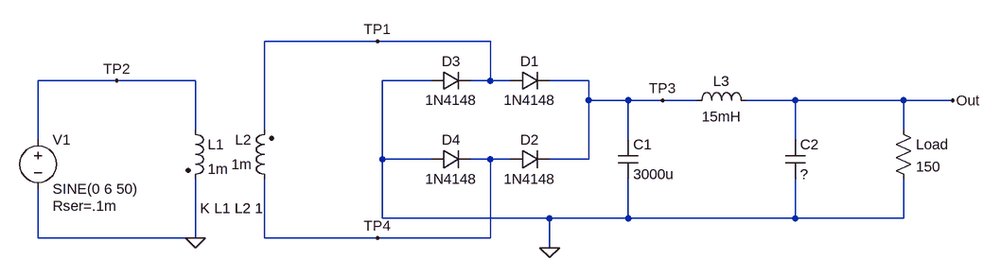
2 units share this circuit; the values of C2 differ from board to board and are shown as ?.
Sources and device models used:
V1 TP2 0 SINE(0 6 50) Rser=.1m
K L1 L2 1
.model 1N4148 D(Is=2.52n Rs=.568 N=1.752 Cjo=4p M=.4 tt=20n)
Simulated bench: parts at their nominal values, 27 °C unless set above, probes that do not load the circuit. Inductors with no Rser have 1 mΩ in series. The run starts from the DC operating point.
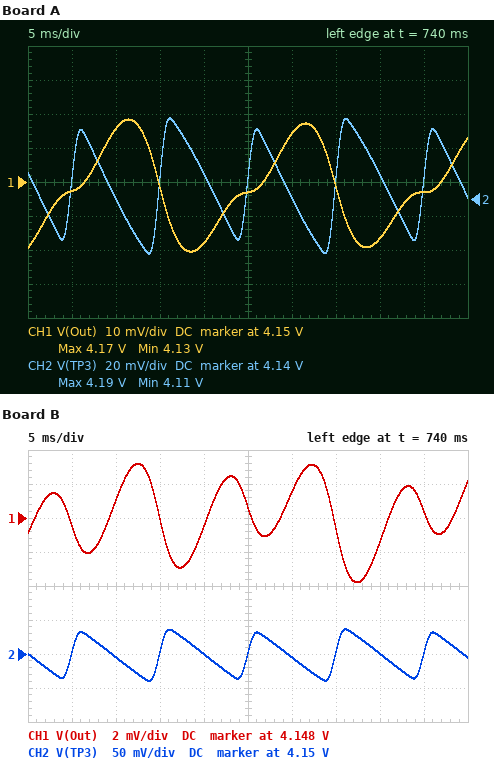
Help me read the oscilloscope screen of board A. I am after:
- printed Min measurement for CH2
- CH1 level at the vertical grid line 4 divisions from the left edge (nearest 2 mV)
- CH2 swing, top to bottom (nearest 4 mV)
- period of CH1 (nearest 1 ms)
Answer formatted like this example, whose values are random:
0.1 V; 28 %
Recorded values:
4.11 V; 4.132 V; 80 mV; 20 ms
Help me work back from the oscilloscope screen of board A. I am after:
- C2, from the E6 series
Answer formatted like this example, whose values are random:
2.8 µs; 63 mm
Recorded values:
1 mF
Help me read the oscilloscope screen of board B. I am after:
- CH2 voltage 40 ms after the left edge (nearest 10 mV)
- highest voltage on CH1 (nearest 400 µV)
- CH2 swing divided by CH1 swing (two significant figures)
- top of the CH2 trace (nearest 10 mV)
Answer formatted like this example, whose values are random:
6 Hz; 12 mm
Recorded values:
4.15 V; 4.1512 V; 11; 4.19 V
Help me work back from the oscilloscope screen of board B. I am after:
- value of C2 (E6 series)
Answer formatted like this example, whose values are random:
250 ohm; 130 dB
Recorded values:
2.2 mF
